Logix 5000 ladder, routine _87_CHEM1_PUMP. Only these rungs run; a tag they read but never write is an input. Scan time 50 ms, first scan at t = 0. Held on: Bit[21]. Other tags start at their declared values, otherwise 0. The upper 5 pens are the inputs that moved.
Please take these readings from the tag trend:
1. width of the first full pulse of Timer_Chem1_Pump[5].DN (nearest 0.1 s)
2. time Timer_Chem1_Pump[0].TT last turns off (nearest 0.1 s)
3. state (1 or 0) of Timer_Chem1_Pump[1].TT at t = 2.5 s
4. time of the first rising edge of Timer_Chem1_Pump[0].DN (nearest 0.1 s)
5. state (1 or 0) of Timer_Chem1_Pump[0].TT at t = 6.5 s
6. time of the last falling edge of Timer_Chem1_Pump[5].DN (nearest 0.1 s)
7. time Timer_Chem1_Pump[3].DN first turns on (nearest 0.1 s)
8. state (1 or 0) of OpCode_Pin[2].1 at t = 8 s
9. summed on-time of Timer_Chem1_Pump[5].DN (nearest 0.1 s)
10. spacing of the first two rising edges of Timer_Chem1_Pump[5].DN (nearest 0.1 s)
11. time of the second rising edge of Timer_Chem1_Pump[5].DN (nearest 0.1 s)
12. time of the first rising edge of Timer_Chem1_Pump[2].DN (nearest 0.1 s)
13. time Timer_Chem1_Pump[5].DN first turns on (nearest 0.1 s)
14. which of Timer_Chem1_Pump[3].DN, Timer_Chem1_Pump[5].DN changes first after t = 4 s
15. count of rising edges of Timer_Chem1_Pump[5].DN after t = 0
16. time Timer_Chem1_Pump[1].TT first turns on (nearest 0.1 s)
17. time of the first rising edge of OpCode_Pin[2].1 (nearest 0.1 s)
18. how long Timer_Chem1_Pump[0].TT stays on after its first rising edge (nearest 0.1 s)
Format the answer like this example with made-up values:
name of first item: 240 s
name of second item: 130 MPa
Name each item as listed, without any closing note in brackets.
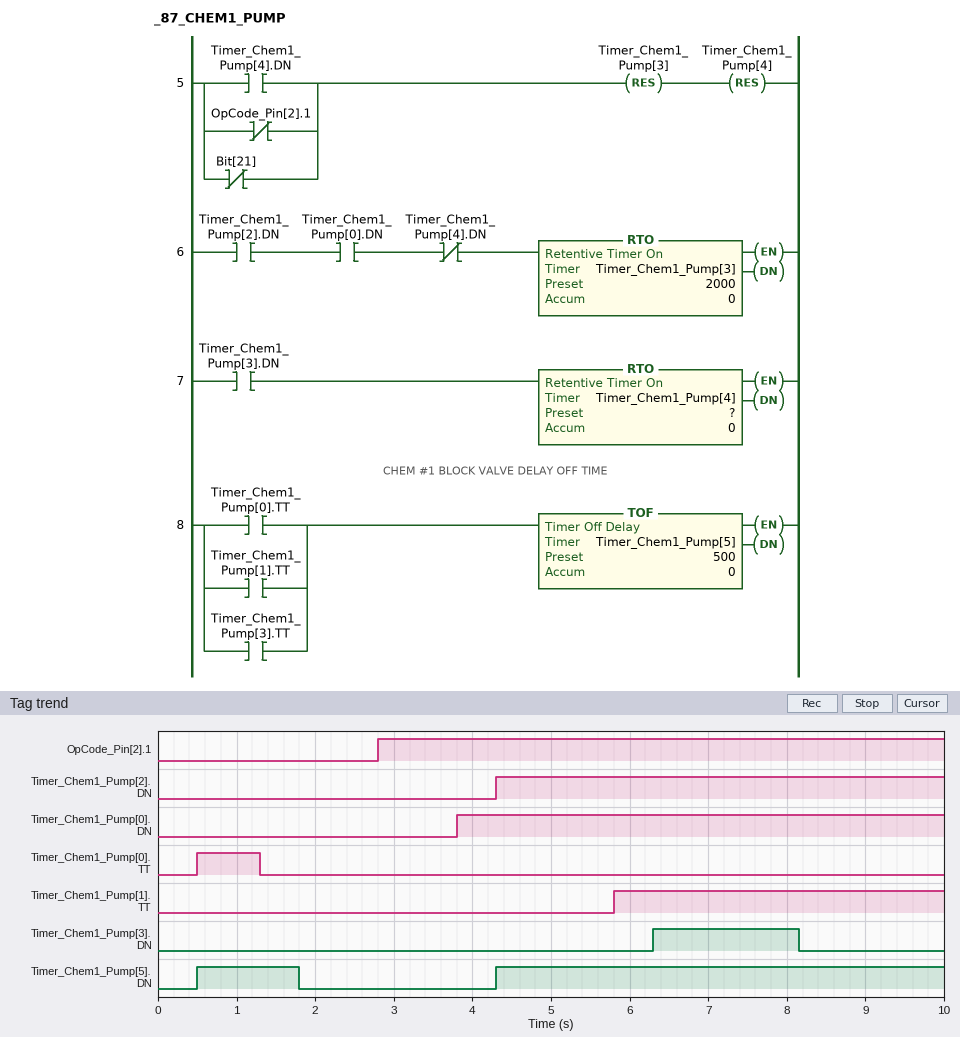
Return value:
width of the first full pulse of Timer_Chem1_Pump[5].DN: 1.3 s
time Timer_Chem1_Pump[0].TT last turns off: 1.3 s
state (1 or 0) of Timer_Chem1_Pump[1].TT at t = 2.5 s: 0
time of the first rising edge of Timer_Chem1_Pump[0].DN: 3.8 s
state (1 or 0) of Timer_Chem1_Pump[0].TT at t = 6.5 s: 0
time of the last falling edge of Timer_Chem1_Pump[5].DN: 1.8 s
time Timer_Chem1_Pump[3].DN first turns on: 6.3 s
state (1 or 0) of OpCode_Pin[2].1 at t = 8 s: 1
summed on-time of Timer_Chem1_Pump[5].DN: 7.0 s
spacing of the first two rising edges of Timer_Chem1_Pump[5].DN: 3.8 s
time of the second rising edge of Timer_Chem1_Pump[5].DN: 4.3 s
time of the first rising edge of Timer_Chem1_Pump[2].DN: 4.3 s
time Timer_Chem1_Pump[5].DN first turns on: 0.5 s
which of Timer_Chem1_Pump[3].DN, Timer_Chem1_Pump[5].DN changes first after t = 4 s: Timer_Chem1_Pump[5].DN
count of rising edges of Timer_Chem1_Pump[5].DN after t = 0: 2
time Timer_Chem1_Pump[1].TT first turns on: 5.8 s
time of the first rising edge of OpCode_Pin[2].1: 2.8 s
how long Timer_Chem1_Pump[0].TT stays on after its first rising edge: 0.8 s
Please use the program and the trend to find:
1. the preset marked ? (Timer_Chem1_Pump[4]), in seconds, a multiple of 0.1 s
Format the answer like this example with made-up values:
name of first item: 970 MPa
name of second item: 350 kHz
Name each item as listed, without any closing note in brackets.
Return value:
the preset marked ? (Timer_Chem1_Pump[4]), in seconds, a multiple of 0.1 s: 1.8 s
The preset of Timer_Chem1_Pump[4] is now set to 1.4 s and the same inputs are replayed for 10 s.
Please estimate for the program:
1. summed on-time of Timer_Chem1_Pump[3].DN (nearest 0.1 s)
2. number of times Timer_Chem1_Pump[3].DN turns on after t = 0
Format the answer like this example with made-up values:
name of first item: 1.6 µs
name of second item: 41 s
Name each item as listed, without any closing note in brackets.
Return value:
summed on-time of Timer_Chem1_Pump[3].DN: 1.7 s
number of times Timer_Chem1_Pump[3].DN turns on after t = 0: 2
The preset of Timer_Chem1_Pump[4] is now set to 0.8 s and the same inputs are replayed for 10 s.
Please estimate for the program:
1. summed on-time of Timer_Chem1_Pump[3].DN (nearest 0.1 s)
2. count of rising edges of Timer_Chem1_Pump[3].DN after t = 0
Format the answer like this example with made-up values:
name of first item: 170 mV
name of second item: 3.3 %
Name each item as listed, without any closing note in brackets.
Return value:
summed on-time of Timer_Chem1_Pump[3].DN: 1.7 s
count of rising edges of Timer_Chem1_Pump[3].DN after t = 0: 2
